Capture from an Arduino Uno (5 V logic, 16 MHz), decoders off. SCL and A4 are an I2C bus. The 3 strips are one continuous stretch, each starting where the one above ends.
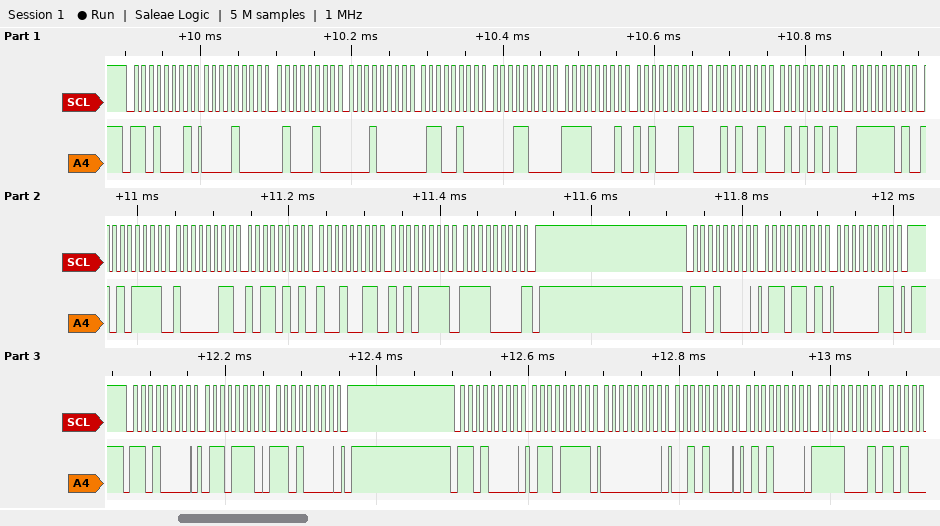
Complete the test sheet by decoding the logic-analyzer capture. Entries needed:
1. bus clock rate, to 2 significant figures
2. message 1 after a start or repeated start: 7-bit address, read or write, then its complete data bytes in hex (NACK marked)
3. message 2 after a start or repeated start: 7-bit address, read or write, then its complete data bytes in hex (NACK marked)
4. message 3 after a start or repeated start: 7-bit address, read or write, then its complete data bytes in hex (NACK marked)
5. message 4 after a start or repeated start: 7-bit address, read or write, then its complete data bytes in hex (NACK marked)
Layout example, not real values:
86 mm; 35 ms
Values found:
100 kHz; 0x68 read: 08 44 10 64 18 F1 A3 29 55 7D AF 83 B5 93 AF F0 NACK; 0x68 write: 6D 03; 0x68 write: 6E D0; 0x68 write: 6F 00 28 50 F1
